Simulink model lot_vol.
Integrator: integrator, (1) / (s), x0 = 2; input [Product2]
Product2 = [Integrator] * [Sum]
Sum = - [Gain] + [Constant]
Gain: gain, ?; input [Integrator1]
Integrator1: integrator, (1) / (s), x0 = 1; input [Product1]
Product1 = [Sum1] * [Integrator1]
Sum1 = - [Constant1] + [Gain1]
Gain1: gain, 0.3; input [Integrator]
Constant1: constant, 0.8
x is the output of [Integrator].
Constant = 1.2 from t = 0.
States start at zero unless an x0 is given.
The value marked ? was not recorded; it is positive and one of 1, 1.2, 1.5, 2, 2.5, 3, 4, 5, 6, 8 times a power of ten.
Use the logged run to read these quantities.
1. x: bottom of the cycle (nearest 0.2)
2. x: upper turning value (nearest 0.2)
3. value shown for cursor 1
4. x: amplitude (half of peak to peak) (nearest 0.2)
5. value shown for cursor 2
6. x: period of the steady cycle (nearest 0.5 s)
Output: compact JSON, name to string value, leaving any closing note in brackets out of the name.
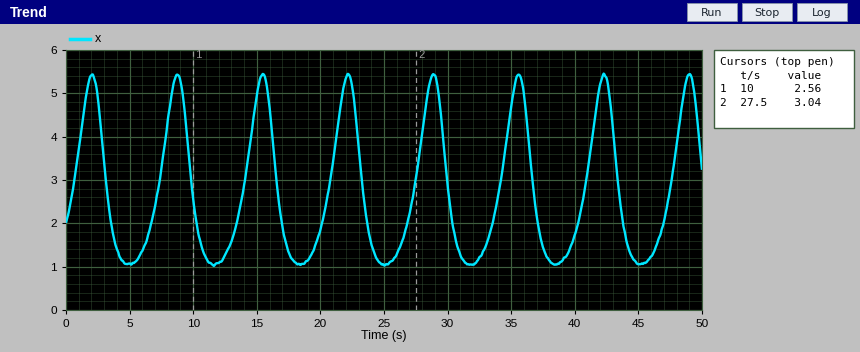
{"x: bottom of the cycle": "1.0", "x: upper turning value": "5.4", "value shown for cursor 1": "2.56", "x: amplitude (half of peak to peak)": "2.2", "value shown for cursor 2": "3.04", "x: period of the steady cycle": "6.5 s"}
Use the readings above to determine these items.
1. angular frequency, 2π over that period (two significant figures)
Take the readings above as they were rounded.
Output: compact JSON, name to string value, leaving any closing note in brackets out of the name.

{"angular frequency, 2π over that period": "0.97 rad/s"}
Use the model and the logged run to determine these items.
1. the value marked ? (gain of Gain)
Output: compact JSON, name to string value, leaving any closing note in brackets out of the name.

{"the value marked ?": "0.6"}
